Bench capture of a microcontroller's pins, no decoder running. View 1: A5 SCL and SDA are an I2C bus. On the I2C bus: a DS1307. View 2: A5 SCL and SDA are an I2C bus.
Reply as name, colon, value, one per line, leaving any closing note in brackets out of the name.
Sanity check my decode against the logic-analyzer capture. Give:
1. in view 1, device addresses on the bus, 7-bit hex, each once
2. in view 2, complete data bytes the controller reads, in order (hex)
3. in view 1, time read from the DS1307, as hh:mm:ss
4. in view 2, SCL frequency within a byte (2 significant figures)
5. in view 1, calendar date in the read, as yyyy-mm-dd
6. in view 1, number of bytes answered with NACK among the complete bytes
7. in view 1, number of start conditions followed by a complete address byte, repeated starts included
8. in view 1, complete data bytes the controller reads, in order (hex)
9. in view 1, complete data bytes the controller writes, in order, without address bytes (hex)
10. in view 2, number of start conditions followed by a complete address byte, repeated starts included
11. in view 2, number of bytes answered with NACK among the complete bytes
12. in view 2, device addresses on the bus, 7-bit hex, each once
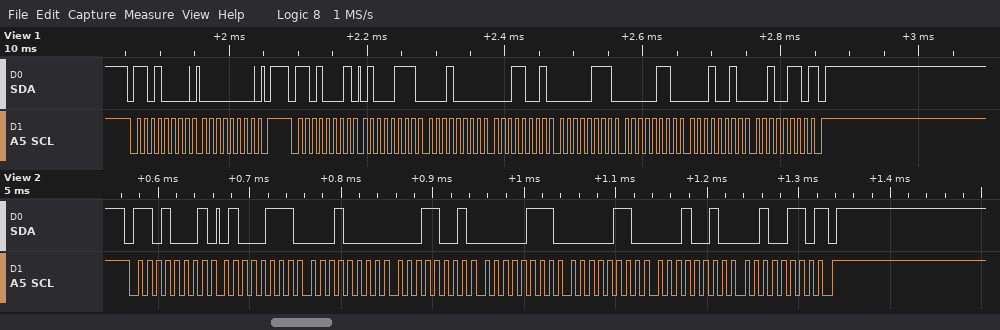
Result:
in view 1, device addresses on the bus, 7-bit hex, each once: 0x68
in view 2, complete data bytes the controller reads, in order: 47 10 19 07 06 12 26
in view 1, time read from the DS1307, as hh:mm:ss: 19:10:47
in view 2, SCL frequency within a byte: 100 kHz
in view 1, calendar date in the read, as yyyy-mm-dd: 2026-12-06
in view 1, number of bytes answered with NACK among the complete bytes: 1
in view 1, number of start conditions followed by a complete address byte, repeated starts included: 2
in view 1, complete data bytes the controller reads, in order: 47 10 19 07 06 12 26
in view 1, complete data bytes the controller writes, in order, without address bytes: 00
in view 2, number of start conditions followed by a complete address byte, repeated starts included: 1
in view 2, number of bytes answered with NACK among the complete bytes: 1
in view 2, device addresses on the bus, 7-bit hex, each once: 0x68
